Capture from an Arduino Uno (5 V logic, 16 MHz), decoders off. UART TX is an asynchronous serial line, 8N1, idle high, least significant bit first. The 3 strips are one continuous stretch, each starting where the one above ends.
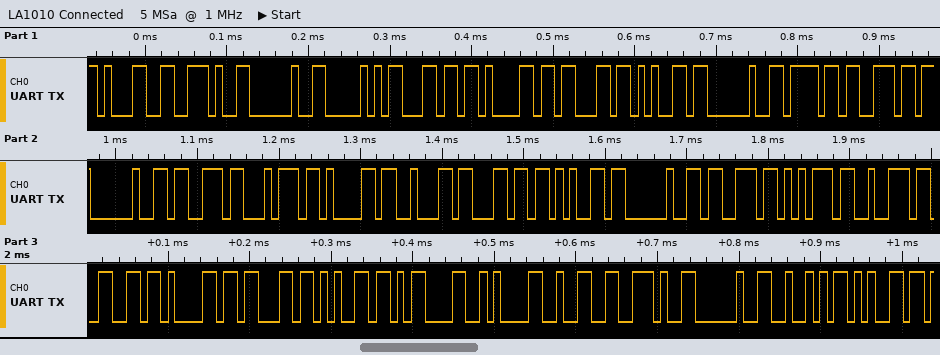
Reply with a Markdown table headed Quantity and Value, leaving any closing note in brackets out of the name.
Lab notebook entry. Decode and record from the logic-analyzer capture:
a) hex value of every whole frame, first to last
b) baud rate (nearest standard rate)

| Quantity | Value |
|---|---|
| hex value of every whole frame, first to last | 31 2E 20 50 6C 61 63 65 20 6F 6E 20 73 74 61 62 6C 65 20 73 75 72 66 61 63 65 0D 0A 32 2E 20 52 65 |
| baud rate | 115200 baud |
